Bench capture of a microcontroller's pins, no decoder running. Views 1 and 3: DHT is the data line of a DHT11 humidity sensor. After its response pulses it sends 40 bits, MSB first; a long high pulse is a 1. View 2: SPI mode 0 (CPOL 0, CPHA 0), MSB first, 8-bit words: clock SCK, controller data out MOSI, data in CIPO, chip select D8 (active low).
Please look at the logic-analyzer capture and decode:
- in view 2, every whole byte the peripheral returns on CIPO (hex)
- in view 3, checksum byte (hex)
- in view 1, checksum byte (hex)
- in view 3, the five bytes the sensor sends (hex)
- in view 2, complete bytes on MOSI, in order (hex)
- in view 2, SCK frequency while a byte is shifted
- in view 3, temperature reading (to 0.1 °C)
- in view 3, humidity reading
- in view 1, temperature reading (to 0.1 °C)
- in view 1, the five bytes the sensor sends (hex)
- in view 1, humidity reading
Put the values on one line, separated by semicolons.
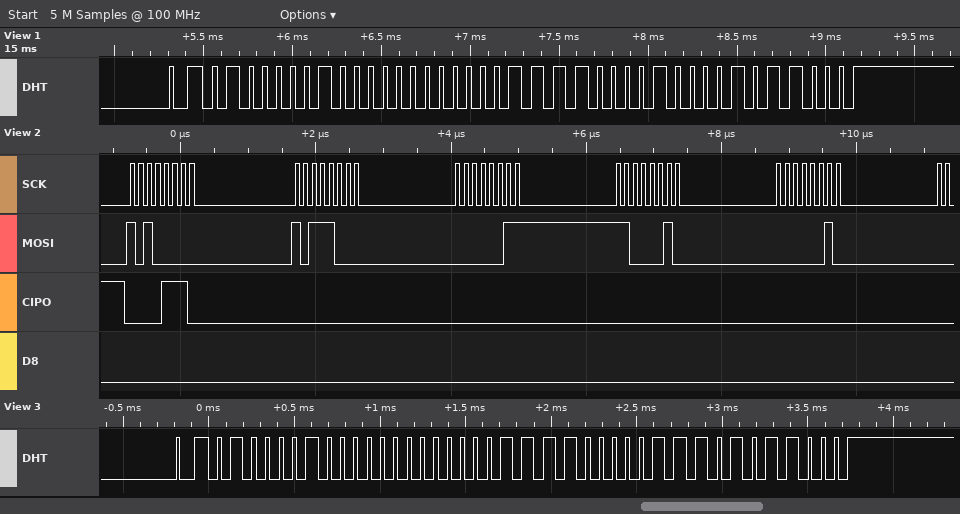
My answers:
0x0E 0x00 0x00 0x00 0x00; 0x58; 0x58; 42 00 0F 07 58; 0xA0 0xB8 0x03 0xC2 0x02; 8 MHz; 15.7 °C; 66 %; 15.8 °C; 41 00 0F 08 58; 65 %
